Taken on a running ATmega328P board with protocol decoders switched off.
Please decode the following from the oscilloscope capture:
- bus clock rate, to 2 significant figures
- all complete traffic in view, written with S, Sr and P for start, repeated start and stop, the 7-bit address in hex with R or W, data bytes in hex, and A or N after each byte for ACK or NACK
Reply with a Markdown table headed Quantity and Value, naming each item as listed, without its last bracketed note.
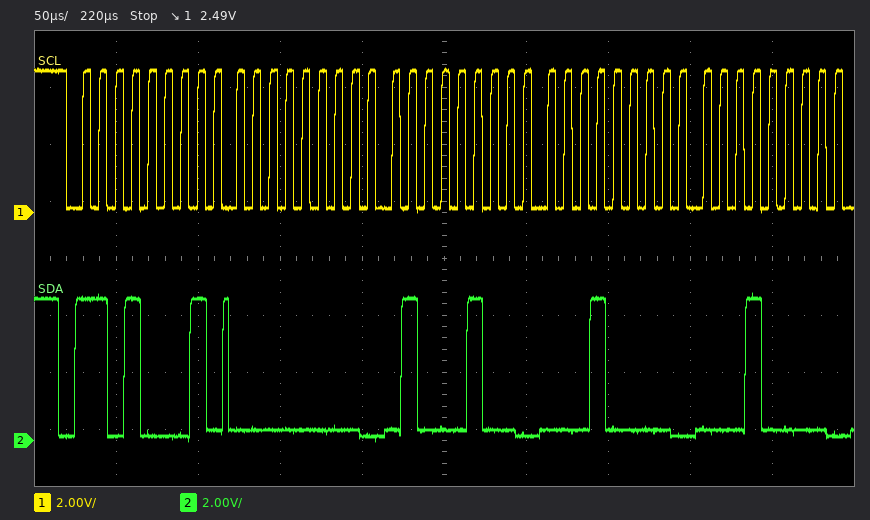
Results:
| Quantity | Value |
|---|---|
| bus clock rate, to 2 significant figures | 100 kHz |
| all complete traffic in view, written with S, Sr and P for start, repeated start and stop, the 7-bit address in hex with R or W, data bytes in hex, and A or N after each byte for ACK or NACK | S 68R A 00 A 44 A 10 A 10 A |
